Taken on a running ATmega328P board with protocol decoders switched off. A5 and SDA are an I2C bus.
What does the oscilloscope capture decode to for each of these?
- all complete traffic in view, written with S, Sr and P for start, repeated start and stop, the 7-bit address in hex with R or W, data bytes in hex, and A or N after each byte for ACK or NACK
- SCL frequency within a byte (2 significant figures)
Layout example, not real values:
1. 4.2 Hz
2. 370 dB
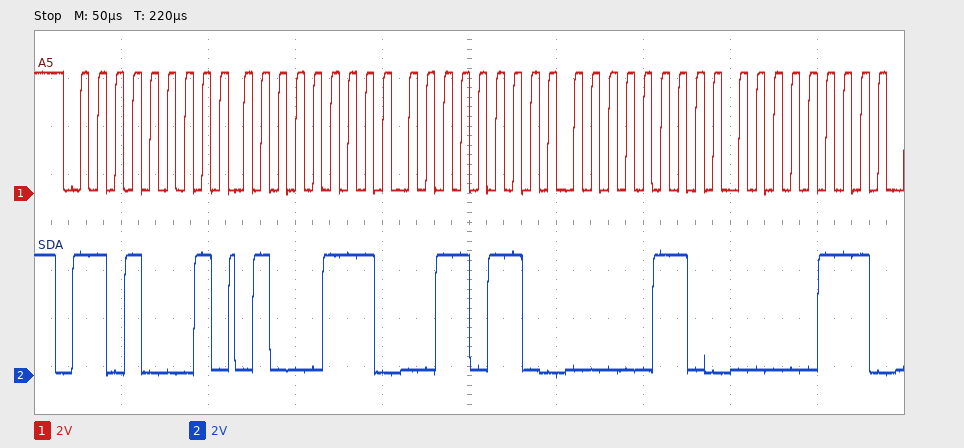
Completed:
1. S 68R A 47 A 36 A 06 A 07 A
2. 100 kHz
